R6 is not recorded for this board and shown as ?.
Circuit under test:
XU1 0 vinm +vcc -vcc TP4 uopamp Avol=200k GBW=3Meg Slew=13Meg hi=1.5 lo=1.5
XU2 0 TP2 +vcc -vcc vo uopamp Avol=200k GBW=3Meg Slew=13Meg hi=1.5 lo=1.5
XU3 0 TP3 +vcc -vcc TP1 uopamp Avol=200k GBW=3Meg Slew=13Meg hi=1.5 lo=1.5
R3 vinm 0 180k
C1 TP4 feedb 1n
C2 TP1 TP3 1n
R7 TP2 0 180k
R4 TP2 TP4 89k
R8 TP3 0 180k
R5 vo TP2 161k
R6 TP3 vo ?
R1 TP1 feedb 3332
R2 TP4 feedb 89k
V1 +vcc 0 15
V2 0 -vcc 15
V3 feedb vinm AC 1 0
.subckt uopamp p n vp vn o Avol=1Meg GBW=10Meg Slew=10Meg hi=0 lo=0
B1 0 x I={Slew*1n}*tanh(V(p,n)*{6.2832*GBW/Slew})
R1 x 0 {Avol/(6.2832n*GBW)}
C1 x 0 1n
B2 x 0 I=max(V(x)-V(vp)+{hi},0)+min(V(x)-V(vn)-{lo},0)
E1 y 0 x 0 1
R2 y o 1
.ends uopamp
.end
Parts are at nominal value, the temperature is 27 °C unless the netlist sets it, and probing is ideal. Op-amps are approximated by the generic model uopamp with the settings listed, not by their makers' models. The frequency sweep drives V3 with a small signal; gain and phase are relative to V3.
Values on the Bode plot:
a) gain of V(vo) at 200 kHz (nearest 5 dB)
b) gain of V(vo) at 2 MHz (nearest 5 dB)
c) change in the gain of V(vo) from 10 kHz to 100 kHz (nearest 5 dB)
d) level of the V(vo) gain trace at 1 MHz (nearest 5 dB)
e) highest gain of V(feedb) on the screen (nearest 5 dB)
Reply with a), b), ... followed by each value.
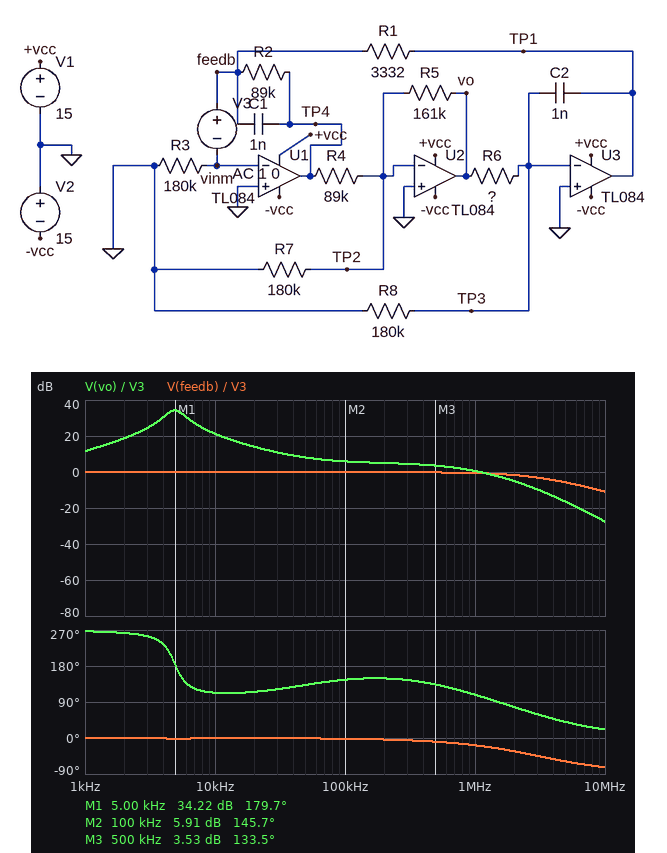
a) 5 dB
b) -5 dB
c) -15 dB
d) 0 dB
e) 0 dB
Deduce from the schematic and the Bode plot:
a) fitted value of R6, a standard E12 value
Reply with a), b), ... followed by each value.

a) 560 kΩ
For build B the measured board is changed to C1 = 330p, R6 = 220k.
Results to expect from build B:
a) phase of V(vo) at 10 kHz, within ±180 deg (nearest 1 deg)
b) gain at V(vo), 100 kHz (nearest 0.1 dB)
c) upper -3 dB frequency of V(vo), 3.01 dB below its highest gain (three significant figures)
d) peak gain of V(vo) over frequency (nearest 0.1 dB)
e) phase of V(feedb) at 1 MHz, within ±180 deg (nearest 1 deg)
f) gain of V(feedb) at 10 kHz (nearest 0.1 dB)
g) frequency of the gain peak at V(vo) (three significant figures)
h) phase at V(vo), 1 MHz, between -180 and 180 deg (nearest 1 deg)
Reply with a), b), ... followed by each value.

a) -118 deg
b) 9.9 dB
c) 16.1 kHz
d) 34.6 dB
e) -18 deg
f) 0.4 dB
g) 13.4 kHz
h) 103 deg
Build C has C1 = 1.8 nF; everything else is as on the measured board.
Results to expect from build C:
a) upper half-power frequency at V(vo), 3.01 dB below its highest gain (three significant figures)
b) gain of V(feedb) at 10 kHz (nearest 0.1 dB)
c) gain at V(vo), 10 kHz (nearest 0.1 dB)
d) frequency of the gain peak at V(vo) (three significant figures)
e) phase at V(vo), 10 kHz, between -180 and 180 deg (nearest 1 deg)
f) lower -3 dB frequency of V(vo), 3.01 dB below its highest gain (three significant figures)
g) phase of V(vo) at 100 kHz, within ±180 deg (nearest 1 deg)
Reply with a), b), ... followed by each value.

a) 4.19 kHz
b) -0.1 dB
c) 15.6 dB
d) 3.68 kHz
e) 115 deg
f) 3.23 kHz
g) 156 deg
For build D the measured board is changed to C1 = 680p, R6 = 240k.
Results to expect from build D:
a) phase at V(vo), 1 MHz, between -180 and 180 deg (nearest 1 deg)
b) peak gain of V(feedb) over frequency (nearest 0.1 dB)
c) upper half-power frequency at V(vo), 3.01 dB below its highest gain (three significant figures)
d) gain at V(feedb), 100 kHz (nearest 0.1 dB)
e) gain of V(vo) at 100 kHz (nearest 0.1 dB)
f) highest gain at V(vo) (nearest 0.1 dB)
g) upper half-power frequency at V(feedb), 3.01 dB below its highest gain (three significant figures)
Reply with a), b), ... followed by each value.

a) 107 deg
b) 0.4 dB
c) 10.4 kHz
d) -0.2 dB
e) 6.8 dB
f) 34.6 dB
g) 2.65 MHz
